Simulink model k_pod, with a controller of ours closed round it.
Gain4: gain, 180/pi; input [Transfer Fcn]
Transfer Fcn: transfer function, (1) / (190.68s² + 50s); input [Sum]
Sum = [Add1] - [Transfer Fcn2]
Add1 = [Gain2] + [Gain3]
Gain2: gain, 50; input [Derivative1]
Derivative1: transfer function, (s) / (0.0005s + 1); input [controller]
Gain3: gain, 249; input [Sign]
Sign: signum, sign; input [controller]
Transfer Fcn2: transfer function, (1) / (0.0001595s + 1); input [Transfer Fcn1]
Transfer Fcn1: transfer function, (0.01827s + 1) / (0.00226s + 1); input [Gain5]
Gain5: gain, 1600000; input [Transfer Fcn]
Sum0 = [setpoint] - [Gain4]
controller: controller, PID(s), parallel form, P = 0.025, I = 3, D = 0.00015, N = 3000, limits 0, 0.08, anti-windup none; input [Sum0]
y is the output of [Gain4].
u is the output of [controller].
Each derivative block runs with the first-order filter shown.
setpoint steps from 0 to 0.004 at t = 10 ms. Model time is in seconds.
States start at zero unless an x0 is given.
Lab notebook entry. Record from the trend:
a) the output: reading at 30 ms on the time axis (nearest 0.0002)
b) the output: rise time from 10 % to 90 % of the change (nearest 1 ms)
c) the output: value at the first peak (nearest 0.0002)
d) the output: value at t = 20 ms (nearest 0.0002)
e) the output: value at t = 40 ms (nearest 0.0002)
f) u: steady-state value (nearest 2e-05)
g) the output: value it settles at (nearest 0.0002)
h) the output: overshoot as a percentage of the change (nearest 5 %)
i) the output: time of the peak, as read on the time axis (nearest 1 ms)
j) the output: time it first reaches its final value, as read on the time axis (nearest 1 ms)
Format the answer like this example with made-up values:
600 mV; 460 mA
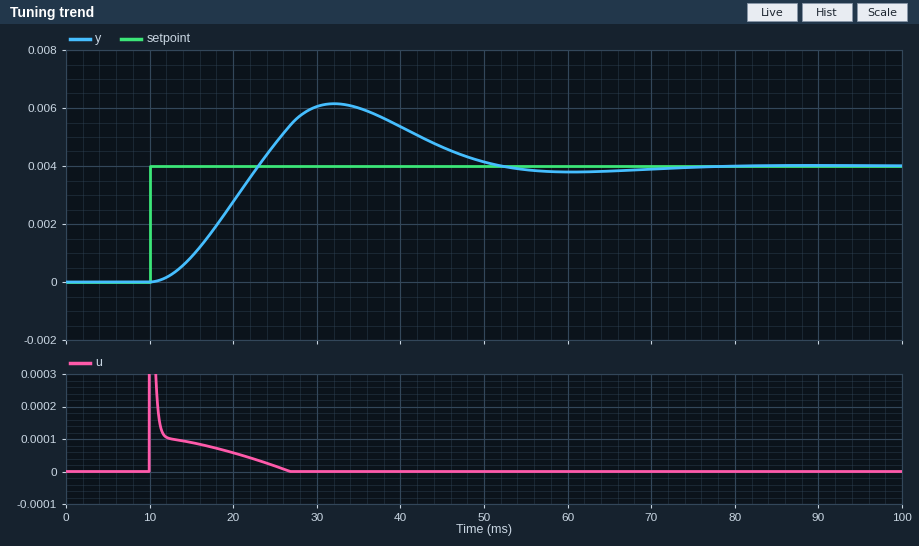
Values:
0.0060; 9 ms; 0.0062; 0.0028; 0.0054; 0.00000; 0.0040; 55 %; 32 ms; 23 ms
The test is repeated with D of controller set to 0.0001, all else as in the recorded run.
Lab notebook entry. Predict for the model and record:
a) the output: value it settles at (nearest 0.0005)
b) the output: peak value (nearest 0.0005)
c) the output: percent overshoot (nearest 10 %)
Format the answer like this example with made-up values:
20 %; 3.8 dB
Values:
0.0040; 0.0065; 60 %
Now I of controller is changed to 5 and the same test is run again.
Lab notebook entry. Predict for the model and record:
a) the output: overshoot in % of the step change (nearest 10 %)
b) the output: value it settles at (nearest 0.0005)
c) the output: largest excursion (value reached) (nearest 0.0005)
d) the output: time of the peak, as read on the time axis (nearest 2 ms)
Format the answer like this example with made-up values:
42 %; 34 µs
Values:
70 %; 0.0040; 0.0070; 34 ms
